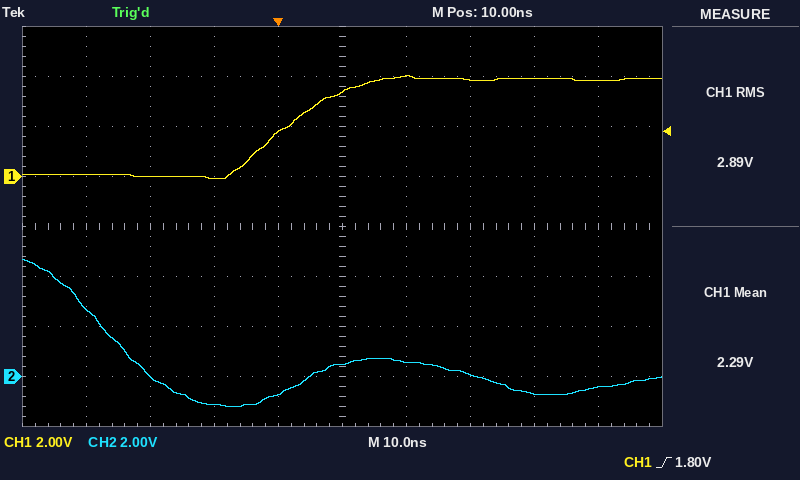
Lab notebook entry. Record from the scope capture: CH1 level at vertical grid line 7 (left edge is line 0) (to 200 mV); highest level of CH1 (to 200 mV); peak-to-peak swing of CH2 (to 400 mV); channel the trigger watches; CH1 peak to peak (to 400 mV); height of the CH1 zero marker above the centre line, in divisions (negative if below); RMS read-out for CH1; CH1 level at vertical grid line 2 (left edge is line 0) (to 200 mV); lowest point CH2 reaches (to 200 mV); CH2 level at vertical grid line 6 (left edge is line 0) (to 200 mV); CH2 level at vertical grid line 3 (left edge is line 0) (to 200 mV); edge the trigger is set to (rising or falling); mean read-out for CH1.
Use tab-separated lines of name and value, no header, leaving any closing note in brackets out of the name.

CH1 level at vertical grid line 7 (left edge is line 0)	3.8 V
highest level of CH1	4.0 V
peak-to-peak swing of CH2	6.0 V
channel the trigger watches	CH1
CH1 peak to peak	4.0 V
height of the CH1 zero marker above the centre line, in divisions	+1.0 div
RMS read-out for CH1	2.89 V
CH1 level at vertical grid line 2 (left edge is line 0)	0.0 V
lowest point CH2 reaches	-1.2 V
CH2 level at vertical grid line 6 (left edge is line 0)	600 mV
CH2 level at vertical grid line 3 (left edge is line 0)	-1.2 V
edge the trigger is set to	rising
mean read-out for CH1	2.29 V
